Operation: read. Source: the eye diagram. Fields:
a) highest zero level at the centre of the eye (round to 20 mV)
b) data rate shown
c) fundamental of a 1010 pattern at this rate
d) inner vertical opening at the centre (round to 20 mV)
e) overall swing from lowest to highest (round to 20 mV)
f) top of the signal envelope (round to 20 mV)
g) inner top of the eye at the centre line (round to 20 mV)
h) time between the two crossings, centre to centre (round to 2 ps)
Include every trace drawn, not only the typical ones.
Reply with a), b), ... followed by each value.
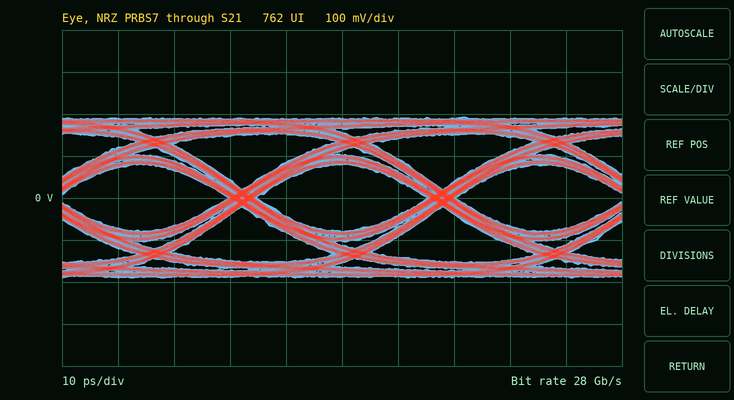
a) -80 mV
b) 28 Gb/s
c) 14 GHz
d) 160 mV
e) 380 mV
f) 200 mV
g) 80 mV
h) 36 ps
